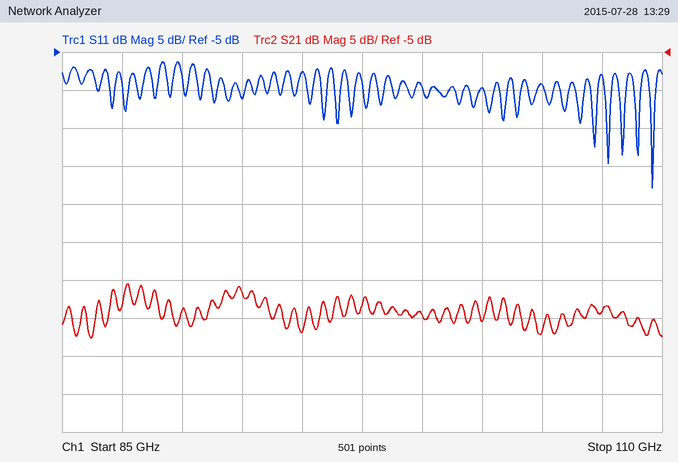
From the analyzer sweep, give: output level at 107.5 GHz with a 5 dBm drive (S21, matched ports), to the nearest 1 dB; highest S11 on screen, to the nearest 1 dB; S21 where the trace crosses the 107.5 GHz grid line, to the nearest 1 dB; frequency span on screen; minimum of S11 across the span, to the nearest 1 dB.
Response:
-34 dBm
-6 dB
-39 dB
25 GHz
-23 dB
